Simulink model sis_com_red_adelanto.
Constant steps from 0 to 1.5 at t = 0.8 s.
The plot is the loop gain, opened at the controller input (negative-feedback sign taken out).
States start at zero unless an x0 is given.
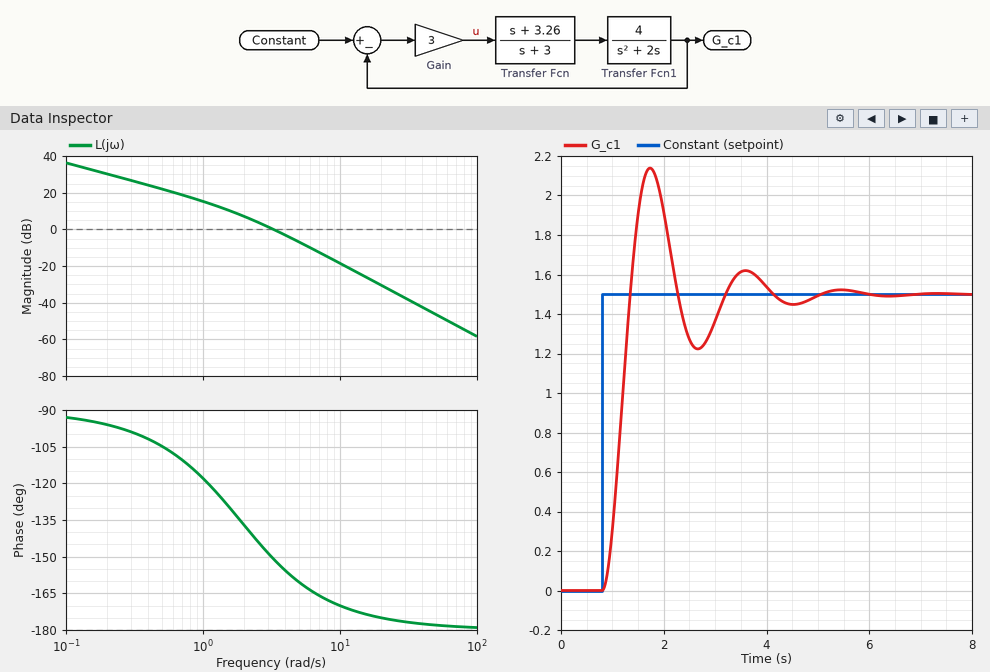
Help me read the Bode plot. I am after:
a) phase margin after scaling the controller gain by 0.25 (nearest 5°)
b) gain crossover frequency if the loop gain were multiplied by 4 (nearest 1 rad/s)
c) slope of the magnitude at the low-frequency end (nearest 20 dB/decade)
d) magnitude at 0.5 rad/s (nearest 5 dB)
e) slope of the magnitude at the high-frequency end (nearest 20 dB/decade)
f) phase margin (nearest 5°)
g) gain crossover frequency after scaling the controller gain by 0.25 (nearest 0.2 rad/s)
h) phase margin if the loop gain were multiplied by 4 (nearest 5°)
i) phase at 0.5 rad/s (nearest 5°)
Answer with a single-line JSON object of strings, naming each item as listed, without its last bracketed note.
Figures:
{"phase margin after scaling the controller gain by 0.25": "55°", "gain crossover frequency if the loop gain were multiplied by 4": "7 rad/s", "slope of the magnitude at the low-frequency end": "-20 dB/decade", "magnitude at 0.5 rad/s": "20 dB", "slope of the magnitude at the high-frequency end": "-40 dB/decade", "phase margin": "30°", "gain crossover frequency after scaling the controller gain by 0.25": "1.4 rad/s", "phase margin if the loop gain were multiplied by 4": "15°", "phase at 0.5 rad/s": "-105°"}
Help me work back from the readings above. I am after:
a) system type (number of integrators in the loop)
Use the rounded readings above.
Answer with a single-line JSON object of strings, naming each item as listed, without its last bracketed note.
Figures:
{"system type": "1"}
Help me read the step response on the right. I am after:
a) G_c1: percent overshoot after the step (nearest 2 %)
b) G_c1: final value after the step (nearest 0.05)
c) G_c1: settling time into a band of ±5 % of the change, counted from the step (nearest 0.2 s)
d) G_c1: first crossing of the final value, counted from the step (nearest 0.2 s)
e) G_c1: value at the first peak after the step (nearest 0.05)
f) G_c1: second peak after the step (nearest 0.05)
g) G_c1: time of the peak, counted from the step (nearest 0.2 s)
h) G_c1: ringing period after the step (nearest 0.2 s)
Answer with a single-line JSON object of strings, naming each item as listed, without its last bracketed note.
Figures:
{"G_c1: percent overshoot after the step": "42 %", "G_c1: final value after the step": "1.50", "G_c1: settling time into a band of ±5 % of the change, counted from the step": "3.0 s", "G_c1: first crossing of the final value, counted from the step": "0.6 s", "G_c1: value at the first peak after the step": "2.15", "G_c1: second peak after the step": "1.60", "G_c1: time of the peak, counted from the step": "1.0 s", "G_c1: ringing period after the step": "1.8 s"}
